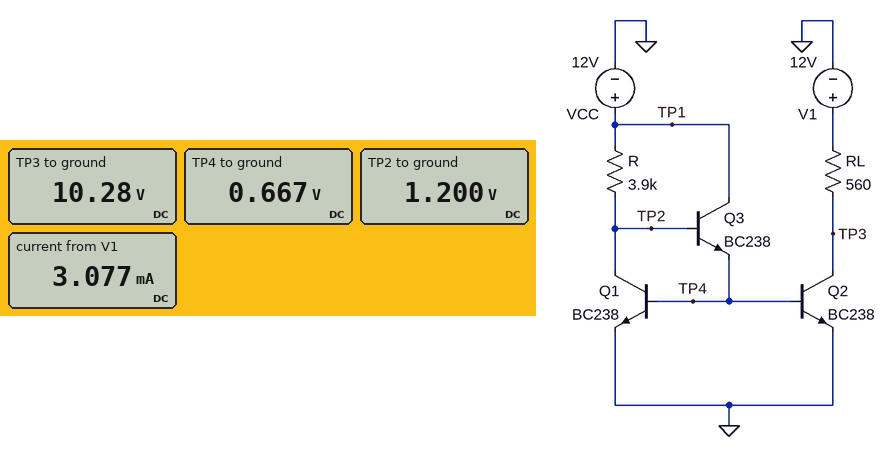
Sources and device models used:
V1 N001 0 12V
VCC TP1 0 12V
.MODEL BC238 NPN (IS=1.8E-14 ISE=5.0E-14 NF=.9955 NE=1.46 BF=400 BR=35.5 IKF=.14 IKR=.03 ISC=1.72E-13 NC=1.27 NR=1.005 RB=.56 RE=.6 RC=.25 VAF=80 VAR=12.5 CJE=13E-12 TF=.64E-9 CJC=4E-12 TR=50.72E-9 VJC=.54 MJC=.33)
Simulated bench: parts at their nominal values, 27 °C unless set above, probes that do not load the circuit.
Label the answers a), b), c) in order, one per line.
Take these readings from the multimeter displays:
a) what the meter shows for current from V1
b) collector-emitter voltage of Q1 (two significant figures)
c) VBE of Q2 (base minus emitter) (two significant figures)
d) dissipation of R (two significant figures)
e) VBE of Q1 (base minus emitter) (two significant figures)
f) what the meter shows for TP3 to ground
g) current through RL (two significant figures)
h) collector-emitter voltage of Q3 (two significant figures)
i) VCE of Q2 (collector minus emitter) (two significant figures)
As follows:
a) 3.077 mA
b) 1.2 V
c) 670 mV
d) 30 mW
e) 670 mV
f) 10.28 V
g) 3.1 mA
h) 11 V
i) 10 V
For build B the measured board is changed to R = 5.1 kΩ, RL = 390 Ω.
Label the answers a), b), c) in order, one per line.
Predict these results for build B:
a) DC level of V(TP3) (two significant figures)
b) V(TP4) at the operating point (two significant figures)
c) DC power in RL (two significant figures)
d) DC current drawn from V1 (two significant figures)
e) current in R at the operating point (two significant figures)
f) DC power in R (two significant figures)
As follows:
a) 11 V
b) 660 mV
c) 2.2 mW
d) 2.4 mA
e) 2.1 mA
f) 23 mW
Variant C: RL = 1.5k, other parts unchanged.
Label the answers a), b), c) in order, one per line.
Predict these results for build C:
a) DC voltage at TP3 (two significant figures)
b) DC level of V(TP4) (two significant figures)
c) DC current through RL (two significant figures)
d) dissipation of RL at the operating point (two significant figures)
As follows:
a) 7.5 V
b) 670 mV
c) 3.0 mA
d) 13 mW
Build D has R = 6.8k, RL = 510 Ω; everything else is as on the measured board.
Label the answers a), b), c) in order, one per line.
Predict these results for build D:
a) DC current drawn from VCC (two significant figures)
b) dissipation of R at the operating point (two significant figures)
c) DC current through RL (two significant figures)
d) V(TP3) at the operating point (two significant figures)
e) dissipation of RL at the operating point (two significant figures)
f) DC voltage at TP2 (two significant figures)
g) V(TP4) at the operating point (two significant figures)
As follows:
a) 1.6 mA
b) 17 mW
c) 1.8 mA
d) 11 V
e) 1.6 mW
f) 1.2 V
g) 650 mV
